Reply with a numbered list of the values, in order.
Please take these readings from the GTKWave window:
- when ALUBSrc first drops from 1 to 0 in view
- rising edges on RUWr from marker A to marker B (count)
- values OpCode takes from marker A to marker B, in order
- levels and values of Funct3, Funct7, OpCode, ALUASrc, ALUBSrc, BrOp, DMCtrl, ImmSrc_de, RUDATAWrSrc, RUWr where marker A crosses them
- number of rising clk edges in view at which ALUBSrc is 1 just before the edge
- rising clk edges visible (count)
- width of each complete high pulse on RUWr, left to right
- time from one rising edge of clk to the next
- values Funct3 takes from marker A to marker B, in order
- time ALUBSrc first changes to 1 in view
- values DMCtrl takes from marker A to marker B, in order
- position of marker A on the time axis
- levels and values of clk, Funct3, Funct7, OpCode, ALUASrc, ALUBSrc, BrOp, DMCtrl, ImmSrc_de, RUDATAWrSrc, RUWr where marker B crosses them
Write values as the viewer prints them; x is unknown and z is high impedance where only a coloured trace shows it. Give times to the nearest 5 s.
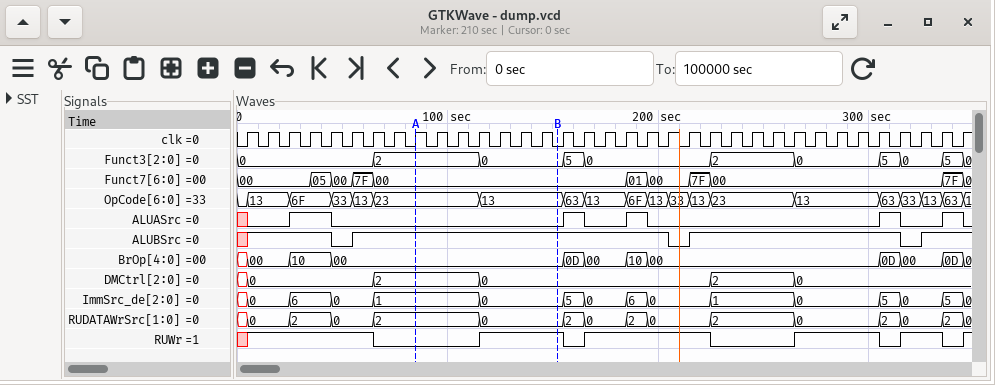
1. 45 s
2. 1
3. 23, 13
4. Funct3=2, Funct7=00, OpCode=23, ALUASrc=0, ALUBSrc=1, BrOp=00, DMCtrl=2, ImmSrc_de=1, RUDATAWrSrc=2, RUWr=0
5. 31
6. 35
7. 40 s, 60 s, 40 s, 20 s
8. 10 s
9. 2, 0
10. 5 s
11. 2, 0
12. 85 s
13. clk=0, Funct3=0, Funct7=00, OpCode=13, ALUASrc=0, ALUBSrc=1, BrOp=00, DMCtrl=0, ImmSrc_de=0, RUDATAWrSrc=0, RUWr=1
